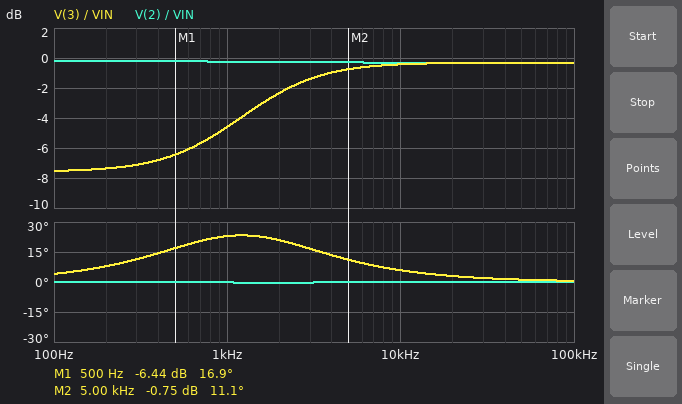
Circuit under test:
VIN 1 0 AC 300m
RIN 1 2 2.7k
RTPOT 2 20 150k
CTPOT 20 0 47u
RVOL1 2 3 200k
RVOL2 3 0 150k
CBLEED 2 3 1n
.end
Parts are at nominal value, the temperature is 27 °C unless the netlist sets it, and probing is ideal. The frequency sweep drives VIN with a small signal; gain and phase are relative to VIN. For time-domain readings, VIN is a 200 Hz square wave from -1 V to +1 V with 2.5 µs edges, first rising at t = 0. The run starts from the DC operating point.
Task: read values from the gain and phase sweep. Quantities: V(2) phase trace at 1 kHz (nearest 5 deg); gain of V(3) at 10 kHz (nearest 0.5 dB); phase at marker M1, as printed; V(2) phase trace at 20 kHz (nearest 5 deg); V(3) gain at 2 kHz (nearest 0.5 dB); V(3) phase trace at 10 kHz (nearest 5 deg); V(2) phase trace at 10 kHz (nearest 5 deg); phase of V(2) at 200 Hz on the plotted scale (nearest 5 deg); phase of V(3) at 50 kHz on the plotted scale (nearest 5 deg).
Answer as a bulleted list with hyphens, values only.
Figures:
- 0 deg
- -0.5 dB
- 16.9 deg
- 0 deg
- -2.5 dB
- 5 deg
- 0 deg
- 0 deg
- 0 deg
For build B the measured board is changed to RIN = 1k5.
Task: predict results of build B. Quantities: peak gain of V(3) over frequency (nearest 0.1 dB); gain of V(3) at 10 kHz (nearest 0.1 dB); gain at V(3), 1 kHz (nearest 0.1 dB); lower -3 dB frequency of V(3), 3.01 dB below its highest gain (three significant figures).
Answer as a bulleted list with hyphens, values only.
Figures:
- -0.2 dB
- -0.3 dB
- -4.5 dB
- 1.46 kHz
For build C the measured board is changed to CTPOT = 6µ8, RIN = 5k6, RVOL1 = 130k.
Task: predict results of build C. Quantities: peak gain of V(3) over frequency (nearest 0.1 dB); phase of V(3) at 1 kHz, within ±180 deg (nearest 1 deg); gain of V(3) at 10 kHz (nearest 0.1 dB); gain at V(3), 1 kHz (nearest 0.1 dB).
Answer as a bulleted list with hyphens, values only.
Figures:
- -0.6 dB
- 15 deg
- -0.8 dB
- -4.5 dB
